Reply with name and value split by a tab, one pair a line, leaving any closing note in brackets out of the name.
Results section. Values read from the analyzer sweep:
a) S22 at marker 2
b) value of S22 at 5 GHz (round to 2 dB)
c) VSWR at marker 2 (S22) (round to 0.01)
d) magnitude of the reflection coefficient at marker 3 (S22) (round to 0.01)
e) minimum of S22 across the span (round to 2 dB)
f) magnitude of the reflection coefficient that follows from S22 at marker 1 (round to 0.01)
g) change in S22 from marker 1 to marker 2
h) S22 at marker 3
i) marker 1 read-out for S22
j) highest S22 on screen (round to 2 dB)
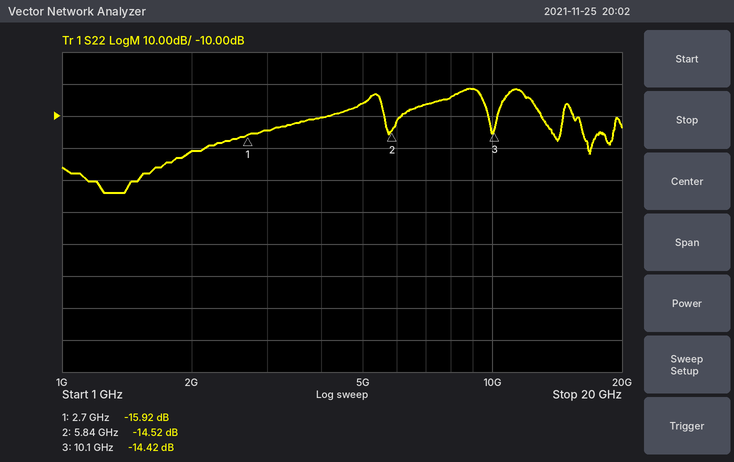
S22 at marker 2	-14.52 dB
value of S22 at 5 GHz	-6 dB
VSWR at marker 2 (S22)	1.46
magnitude of the reflection coefficient at marker 3 (S22)	0.19
minimum of S22 across the span	-34 dB
magnitude of the reflection coefficient that follows from S22 at marker 1	0.16
change in S22 from marker 1 to marker 2	1.40 dB
S22 at marker 3	-14.42 dB
marker 1 read-out for S22	-15.92 dB
highest S22 on screen	-2 dB
